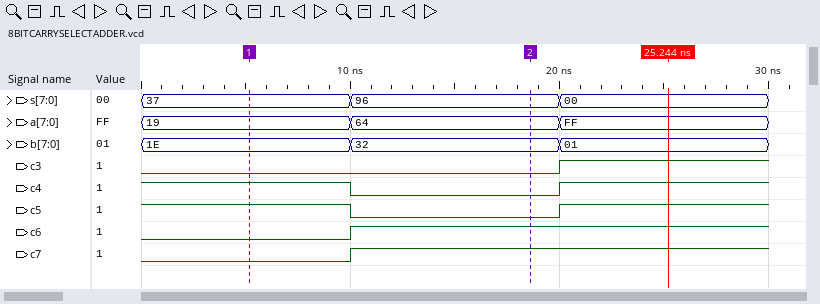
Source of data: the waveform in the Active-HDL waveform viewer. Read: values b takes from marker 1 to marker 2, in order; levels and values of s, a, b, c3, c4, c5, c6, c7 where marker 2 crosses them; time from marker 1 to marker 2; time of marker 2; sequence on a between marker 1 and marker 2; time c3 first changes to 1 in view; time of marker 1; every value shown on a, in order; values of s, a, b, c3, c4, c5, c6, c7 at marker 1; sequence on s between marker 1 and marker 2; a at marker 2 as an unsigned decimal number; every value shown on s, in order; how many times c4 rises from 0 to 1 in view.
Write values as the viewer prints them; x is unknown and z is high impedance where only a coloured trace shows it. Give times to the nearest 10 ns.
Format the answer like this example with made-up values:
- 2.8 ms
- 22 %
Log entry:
- 1E, 32
- s=96, a=64, b=32, c3=0, c4=0, c5=0, c6=1, c7=1
- 10 ns
- 20 ns
- 19, 64
- 20 ns
- 10 ns
- 19, 64, FF
- s=37, a=19, b=1E, c3=0, c4=1, c5=1, c6=0, c7=0
- 37, 96
- 100
- 37, 96, 00
- 1
